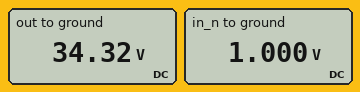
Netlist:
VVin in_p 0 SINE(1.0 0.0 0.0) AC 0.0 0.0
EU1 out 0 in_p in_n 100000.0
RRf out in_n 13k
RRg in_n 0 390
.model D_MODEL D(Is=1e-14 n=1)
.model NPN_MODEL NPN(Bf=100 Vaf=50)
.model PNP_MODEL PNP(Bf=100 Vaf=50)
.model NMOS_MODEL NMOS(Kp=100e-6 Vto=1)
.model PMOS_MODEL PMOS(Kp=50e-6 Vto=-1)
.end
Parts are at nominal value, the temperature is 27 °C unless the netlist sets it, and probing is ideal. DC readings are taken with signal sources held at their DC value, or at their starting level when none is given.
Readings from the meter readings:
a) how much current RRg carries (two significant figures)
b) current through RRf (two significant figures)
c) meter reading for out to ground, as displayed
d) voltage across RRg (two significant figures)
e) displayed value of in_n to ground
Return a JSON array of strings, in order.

["2.6 mA", "2.6 mA", "34.32 V", "1.0 V", "1.000 V"]
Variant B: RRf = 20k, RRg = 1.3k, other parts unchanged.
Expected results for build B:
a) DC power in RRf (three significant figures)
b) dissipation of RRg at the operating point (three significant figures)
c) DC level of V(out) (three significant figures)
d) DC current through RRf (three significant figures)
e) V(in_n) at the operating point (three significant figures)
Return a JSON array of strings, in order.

["11.8 mW", "769 µW", "16.4 V", "769 µA", "1.00 V"]
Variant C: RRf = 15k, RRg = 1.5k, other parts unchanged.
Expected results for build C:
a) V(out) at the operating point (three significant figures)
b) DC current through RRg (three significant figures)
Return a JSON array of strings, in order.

["11.0 V", "667 µA"]
